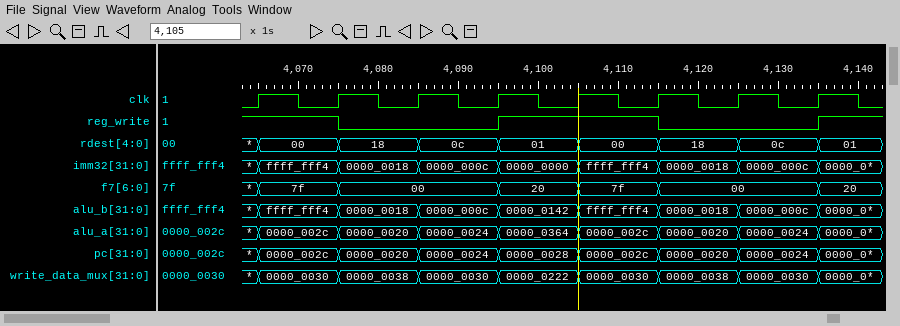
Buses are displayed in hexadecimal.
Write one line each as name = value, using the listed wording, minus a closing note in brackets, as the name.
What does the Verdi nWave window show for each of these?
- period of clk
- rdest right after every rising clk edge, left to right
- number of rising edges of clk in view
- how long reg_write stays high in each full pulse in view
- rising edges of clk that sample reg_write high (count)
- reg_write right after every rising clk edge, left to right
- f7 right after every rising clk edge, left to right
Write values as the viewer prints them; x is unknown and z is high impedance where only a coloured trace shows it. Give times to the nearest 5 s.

period of clk = 10 s
rdest right after every rising clk edge, left to right = 00, 18, 0c, 01, 00, 18, 0c, 01
number of rising edges of clk in view = 8
how long reg_write stays high in each full pulse in view = 20 s
rising edges of clk that sample reg_write high = 4
reg_write right after every rising clk edge, left to right = 1 0 0 1 1 0 0 1
f7 right after every rising clk edge, left to right = 7f, 00, 00, 20, 7f, 00, 00, 20
